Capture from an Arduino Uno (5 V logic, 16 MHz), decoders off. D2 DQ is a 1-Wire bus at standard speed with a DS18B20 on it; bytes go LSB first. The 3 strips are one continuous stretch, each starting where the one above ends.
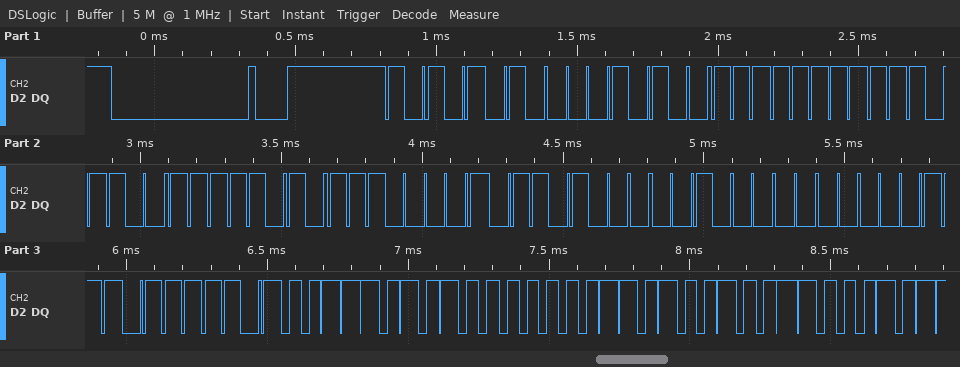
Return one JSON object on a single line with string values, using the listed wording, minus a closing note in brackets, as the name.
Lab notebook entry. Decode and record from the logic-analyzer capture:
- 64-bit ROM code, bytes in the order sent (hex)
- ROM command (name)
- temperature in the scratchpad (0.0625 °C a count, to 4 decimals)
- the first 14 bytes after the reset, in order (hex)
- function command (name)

{"64-bit ROM code, bytes in the order sent": "28 FF 37 5F 87 16 04 E0", "ROM command": "Match ROM", "temperature in the scratchpad": "21.7500 °C", "the first 14 bytes after the reset, in order": "55 28 FF 37 5F 87 16 04 E0 BE 5C 01 4B 46", "function command": "Read Scratchpad"}
